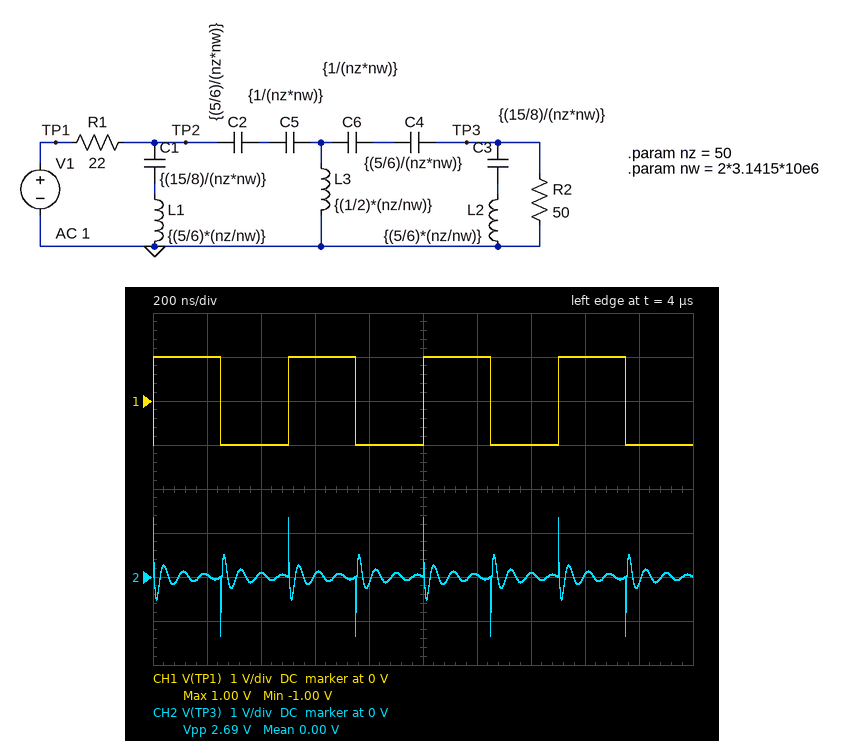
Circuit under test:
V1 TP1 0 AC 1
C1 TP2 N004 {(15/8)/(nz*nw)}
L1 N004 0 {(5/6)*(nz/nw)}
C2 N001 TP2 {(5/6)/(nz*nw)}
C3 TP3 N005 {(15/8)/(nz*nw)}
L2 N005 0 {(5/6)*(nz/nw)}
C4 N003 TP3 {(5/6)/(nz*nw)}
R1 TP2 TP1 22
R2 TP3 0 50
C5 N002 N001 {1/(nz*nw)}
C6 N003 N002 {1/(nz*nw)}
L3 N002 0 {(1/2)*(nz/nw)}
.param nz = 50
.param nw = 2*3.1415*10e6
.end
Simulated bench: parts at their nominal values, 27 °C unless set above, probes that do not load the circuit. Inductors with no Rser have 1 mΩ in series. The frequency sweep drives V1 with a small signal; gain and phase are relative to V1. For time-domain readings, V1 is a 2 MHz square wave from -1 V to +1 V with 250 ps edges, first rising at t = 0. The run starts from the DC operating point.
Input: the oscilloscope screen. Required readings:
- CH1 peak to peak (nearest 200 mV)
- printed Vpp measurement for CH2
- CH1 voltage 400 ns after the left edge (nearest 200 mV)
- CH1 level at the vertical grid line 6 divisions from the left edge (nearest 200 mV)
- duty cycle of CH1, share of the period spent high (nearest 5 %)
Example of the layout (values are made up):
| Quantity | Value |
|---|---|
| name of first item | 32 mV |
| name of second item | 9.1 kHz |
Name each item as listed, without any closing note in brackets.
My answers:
| Quantity | Value |
|---|---|
| CH1 peak to peak | 2.0 V |
| printed Vpp measurement for CH2 | 2.69 V |
| CH1 voltage 400 ns after the left edge | -1.0 V |
| CH1 level at the vertical grid line 6 divisions from the left edge | 1.0 V |
| duty cycle of CH1, share of the period spent high | 50 % |
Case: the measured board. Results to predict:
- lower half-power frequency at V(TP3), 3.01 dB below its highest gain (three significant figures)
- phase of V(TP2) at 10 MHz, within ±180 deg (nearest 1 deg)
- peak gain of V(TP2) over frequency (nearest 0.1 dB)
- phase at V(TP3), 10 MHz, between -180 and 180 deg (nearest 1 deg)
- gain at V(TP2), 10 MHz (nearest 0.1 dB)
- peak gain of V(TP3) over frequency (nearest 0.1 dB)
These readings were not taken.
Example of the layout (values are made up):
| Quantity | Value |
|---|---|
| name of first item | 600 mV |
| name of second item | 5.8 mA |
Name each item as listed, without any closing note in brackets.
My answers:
| Quantity | Value |
|---|---|
| lower half-power frequency at V(TP3), 3.01 dB below its highest gain | 12.4 MHz |
| phase of V(TP2) at 10 MHz, within ±180 deg | 50 deg |
| peak gain of V(TP2) over frequency | 0 dB |
| phase at V(TP3), 10 MHz, between -180 and 180 deg | 29 deg |
| gain at V(TP2), 10 MHz | -3.8 dB |
| peak gain of V(TP3) over frequency | -2.7 dB |
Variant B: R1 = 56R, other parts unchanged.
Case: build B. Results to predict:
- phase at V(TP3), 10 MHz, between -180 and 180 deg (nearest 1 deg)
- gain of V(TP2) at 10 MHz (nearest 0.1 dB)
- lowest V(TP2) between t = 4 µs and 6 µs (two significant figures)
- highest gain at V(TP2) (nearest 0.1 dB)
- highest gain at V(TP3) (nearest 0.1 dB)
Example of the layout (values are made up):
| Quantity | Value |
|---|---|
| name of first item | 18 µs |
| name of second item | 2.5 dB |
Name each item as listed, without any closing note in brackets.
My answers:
| Quantity | Value |
|---|---|
| phase at V(TP3), 10 MHz, between -180 and 180 deg | 51 deg |
| gain of V(TP2) at 10 MHz | -10.0 dB |
| lowest V(TP2) between t = 4 µs and 6 µs | -1.0 V |
| highest gain at V(TP2) | 0 dB |
| highest gain at V(TP3) | -6.5 dB |
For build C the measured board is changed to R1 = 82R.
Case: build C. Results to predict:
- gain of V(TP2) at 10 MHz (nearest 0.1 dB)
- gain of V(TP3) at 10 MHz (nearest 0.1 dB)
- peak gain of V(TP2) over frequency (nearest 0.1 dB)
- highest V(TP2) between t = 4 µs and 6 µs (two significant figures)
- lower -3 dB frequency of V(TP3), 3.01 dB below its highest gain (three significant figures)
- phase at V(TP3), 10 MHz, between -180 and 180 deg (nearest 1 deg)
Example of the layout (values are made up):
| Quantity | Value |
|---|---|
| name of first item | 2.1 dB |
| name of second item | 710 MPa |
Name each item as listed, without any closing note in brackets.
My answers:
| Quantity | Value |
|---|---|
| gain of V(TP2) at 10 MHz | -13.1 dB |
| gain of V(TP3) at 10 MHz | -36.7 dB |
| peak gain of V(TP2) over frequency | 0 dB |
| highest V(TP2) between t = 4 µs and 6 µs | 980 mV |
| lower -3 dB frequency of V(TP3), 3.01 dB below its highest gain | 12.1 MHz |
| phase at V(TP3), 10 MHz, between -180 and 180 deg | 57 deg |
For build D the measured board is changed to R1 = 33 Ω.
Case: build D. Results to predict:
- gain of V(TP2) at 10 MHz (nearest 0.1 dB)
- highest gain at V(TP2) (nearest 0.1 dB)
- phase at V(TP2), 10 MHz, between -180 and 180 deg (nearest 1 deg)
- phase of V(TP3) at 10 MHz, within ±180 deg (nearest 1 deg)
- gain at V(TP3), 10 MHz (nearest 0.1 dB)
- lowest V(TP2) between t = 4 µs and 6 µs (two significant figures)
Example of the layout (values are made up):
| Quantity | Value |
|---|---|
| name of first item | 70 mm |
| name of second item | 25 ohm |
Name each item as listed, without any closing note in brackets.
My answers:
| Quantity | Value |
|---|---|
| gain of V(TP2) at 10 MHz | -6.2 dB |
| highest gain at V(TP2) | 0 dB |
| phase at V(TP2), 10 MHz, between -180 and 180 deg | 60 deg |
| phase of V(TP3) at 10 MHz, within ±180 deg | 40 deg |
| gain at V(TP3), 10 MHz | -29.8 dB |
| lowest V(TP2) between t = 4 µs and 6 µs | -1.2 V |
